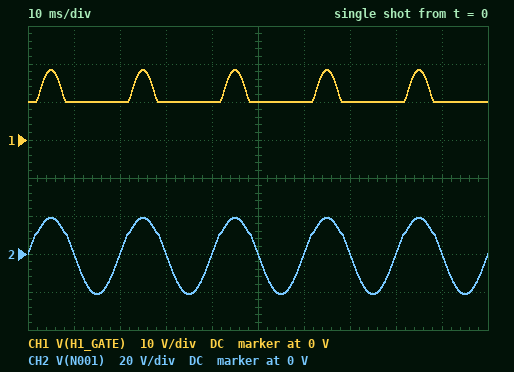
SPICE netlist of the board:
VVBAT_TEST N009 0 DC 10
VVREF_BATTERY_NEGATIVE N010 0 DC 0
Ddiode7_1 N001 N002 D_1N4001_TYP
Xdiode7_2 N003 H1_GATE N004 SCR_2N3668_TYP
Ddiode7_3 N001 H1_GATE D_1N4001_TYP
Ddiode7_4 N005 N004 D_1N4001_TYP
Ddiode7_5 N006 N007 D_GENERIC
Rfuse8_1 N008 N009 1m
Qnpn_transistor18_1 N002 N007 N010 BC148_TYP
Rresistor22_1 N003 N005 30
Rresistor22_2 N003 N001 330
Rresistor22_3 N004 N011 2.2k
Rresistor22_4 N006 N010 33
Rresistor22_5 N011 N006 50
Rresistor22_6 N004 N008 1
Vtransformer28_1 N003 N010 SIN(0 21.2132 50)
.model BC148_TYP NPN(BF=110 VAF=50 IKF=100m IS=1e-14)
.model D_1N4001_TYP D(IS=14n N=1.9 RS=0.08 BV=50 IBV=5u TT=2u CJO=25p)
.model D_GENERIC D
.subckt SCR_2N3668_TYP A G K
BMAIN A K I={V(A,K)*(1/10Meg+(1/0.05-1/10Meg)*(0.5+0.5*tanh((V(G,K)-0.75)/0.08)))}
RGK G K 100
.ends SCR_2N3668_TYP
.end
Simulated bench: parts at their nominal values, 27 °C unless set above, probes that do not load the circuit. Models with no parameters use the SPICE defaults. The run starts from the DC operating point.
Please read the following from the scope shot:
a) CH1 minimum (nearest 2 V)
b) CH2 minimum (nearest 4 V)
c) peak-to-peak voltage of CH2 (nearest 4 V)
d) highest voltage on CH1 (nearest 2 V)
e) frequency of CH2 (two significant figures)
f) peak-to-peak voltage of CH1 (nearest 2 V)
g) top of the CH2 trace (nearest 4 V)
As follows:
10 V
-20 V
40 V
18 V
50 Hz
8 V
20 V
